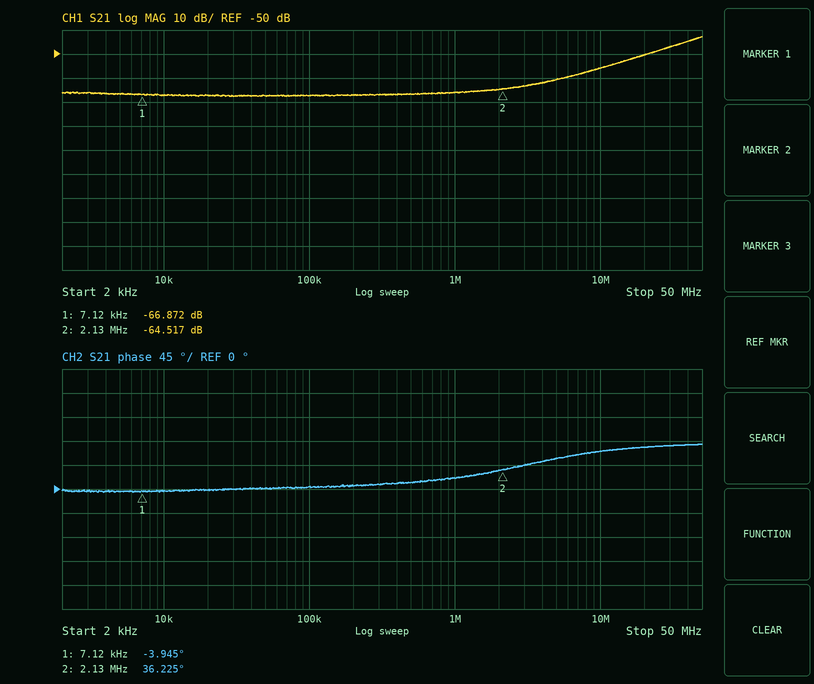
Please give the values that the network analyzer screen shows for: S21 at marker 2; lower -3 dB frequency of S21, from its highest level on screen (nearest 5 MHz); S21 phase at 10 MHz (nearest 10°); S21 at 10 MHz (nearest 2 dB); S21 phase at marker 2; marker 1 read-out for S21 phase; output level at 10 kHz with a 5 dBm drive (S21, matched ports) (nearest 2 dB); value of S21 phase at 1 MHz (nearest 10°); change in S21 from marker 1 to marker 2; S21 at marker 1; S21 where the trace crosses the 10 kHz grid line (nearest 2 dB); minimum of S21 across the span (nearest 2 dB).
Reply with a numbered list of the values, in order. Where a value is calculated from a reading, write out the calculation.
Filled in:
1. -64.517 dB
2. 35 MHz
3. 70°
4. -56 dB
5. 36.225°
6. -3.945°
7. 5 dBm + (-68 dB) = -62 dBm
8. 20°
9. -64.517 − (-66.872) = 2.355 dB
10. -66.872 dB
11. -68 dB
12. -68 dB
